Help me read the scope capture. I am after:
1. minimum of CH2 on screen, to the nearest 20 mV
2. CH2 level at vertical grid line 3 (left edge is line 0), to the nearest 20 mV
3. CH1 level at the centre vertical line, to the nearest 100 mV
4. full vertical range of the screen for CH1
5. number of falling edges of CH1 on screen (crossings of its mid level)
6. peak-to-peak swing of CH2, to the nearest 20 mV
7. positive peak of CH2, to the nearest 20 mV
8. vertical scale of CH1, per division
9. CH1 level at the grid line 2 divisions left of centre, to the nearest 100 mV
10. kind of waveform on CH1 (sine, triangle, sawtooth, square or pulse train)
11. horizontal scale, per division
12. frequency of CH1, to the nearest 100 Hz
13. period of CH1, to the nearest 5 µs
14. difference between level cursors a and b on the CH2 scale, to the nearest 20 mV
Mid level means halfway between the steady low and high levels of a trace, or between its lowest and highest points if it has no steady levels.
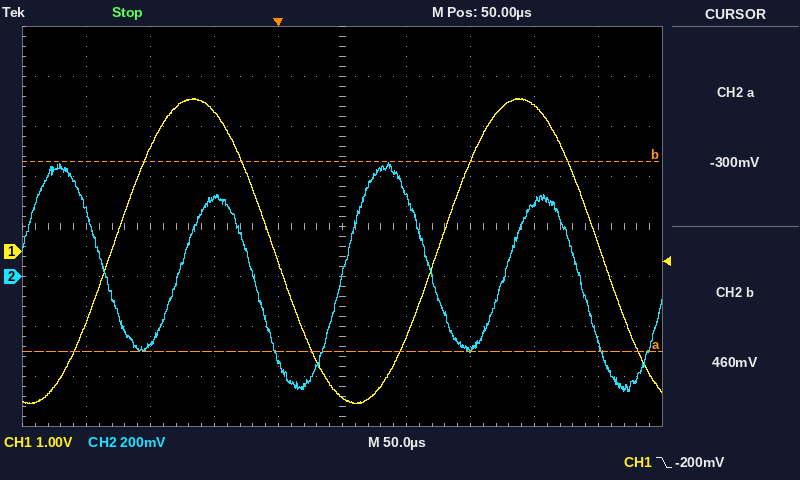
-460 mV
320 mV
-2.9 V
8 V
2
920 mV
460 mV
1 V
2.8 V
sine
50 µs
3.9 kHz
255 µs
760 mV
